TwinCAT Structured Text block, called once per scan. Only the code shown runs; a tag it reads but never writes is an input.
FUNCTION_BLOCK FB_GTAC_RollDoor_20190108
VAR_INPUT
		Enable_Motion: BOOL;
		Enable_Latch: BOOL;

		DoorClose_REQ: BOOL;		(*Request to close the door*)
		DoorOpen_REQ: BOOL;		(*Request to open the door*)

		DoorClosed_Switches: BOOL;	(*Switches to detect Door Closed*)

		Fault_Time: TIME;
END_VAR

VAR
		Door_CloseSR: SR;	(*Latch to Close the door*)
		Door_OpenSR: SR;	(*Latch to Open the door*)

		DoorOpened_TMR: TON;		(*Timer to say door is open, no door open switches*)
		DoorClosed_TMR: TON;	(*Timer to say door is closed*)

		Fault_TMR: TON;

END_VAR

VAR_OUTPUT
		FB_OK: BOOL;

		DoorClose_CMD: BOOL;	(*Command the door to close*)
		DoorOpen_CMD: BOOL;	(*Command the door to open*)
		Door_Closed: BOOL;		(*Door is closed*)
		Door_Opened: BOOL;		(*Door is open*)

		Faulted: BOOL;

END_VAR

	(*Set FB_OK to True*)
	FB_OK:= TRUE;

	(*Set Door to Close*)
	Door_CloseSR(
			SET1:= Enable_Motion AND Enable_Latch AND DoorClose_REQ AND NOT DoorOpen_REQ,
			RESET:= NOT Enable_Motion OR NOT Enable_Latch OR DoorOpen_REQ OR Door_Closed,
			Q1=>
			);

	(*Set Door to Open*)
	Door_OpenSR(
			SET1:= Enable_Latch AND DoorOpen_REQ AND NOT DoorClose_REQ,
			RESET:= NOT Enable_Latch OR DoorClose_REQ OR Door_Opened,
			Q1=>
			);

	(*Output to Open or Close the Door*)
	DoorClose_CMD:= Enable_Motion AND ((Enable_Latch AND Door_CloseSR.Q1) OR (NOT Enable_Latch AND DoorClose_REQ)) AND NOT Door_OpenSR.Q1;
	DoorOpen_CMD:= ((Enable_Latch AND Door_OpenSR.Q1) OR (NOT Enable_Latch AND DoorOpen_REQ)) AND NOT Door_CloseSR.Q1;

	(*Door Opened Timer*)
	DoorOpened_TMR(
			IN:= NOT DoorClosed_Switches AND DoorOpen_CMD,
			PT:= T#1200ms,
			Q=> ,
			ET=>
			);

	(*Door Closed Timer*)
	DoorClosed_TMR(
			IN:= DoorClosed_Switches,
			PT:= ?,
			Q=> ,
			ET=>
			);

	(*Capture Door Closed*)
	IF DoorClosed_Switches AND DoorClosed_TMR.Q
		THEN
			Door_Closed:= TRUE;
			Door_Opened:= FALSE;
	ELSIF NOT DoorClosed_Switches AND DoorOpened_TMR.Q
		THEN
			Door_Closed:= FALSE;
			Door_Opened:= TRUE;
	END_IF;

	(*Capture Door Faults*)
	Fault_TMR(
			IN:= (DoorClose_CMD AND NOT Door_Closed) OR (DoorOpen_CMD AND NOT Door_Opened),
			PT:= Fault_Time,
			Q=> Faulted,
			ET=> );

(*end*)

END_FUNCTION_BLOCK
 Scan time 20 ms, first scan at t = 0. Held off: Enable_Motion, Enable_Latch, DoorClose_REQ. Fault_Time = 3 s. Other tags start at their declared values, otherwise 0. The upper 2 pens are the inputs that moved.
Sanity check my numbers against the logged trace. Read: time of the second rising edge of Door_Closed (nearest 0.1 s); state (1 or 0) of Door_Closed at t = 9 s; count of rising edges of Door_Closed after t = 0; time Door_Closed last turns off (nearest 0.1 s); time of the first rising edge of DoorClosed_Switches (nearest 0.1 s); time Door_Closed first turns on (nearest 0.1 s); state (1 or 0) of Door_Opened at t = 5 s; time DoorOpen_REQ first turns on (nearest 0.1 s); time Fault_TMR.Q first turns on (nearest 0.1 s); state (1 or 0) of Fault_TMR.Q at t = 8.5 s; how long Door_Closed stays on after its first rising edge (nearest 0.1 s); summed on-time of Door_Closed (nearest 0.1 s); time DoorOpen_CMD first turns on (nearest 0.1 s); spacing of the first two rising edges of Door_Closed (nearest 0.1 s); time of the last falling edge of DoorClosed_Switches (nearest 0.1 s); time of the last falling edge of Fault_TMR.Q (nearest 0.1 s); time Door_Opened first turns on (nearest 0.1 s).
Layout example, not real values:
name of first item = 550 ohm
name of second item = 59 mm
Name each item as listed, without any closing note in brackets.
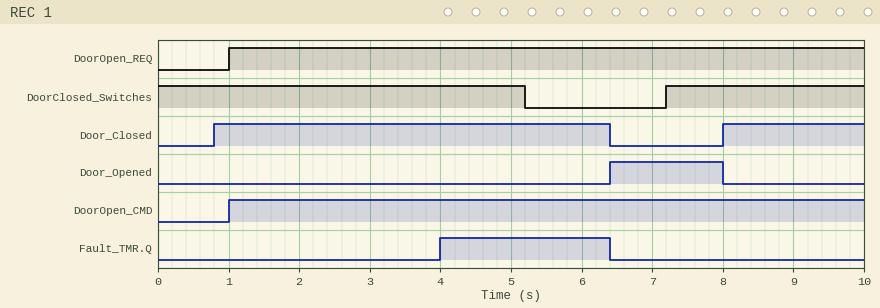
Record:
time of the second rising edge of Door_Closed = 8.0 s
state (1 or 0) of Door_Closed at t = 9 s = 1
count of rising edges of Door_Closed after t = 0 = 2
time Door_Closed last turns off = 6.4 s
time of the first rising edge of DoorClosed_Switches = 7.2 s
time Door_Closed first turns on = 0.8 s
state (1 or 0) of Door_Opened at t = 5 s = 0
time DoorOpen_REQ first turns on = 1.0 s
time Fault_TMR.Q first turns on = 4.0 s
state (1 or 0) of Fault_TMR.Q at t = 8.5 s = 0
how long Door_Closed stays on after its first rising edge = 5.6 s
summed on-time of Door_Closed = 7.6 s
time DoorOpen_CMD first turns on = 1.0 s
spacing of the first two rising edges of Door_Closed = 7.2 s
time of the last falling edge of DoorClosed_Switches = 5.2 s
time of the last falling edge of Fault_TMR.Q = 6.4 s
time Door_Opened first turns on = 6.4 s
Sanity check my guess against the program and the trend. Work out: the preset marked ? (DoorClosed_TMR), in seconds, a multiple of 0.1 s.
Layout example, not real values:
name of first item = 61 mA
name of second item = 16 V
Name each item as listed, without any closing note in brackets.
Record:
the preset marked ? (DoorClosed_TMR), in seconds, a multiple of 0.1 s = 0.8 s
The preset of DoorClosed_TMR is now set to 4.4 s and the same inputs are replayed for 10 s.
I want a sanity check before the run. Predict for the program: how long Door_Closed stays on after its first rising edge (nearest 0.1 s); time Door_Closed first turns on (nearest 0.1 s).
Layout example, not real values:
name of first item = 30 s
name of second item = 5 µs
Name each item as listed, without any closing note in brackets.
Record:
how long Door_Closed stays on after its first rising edge = 2.0 s
time Door_Closed first turns on = 4.4 s
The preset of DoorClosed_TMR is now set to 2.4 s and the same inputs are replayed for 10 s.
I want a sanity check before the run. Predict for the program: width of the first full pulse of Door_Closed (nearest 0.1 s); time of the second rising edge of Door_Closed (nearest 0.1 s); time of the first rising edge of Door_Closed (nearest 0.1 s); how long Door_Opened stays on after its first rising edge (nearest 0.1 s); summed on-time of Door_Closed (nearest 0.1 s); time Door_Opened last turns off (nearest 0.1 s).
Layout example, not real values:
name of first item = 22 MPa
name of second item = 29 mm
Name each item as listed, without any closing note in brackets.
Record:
width of the first full pulse of Door_Closed = 4.0 s
time of the second rising edge of Door_Closed = 9.6 s
time of the first rising edge of Door_Closed = 2.4 s
how long Door_Opened stays on after its first rising edge = 3.2 s
summed on-time of Door_Closed = 4.4 s
time Door_Opened last turns off = 9.6 s
